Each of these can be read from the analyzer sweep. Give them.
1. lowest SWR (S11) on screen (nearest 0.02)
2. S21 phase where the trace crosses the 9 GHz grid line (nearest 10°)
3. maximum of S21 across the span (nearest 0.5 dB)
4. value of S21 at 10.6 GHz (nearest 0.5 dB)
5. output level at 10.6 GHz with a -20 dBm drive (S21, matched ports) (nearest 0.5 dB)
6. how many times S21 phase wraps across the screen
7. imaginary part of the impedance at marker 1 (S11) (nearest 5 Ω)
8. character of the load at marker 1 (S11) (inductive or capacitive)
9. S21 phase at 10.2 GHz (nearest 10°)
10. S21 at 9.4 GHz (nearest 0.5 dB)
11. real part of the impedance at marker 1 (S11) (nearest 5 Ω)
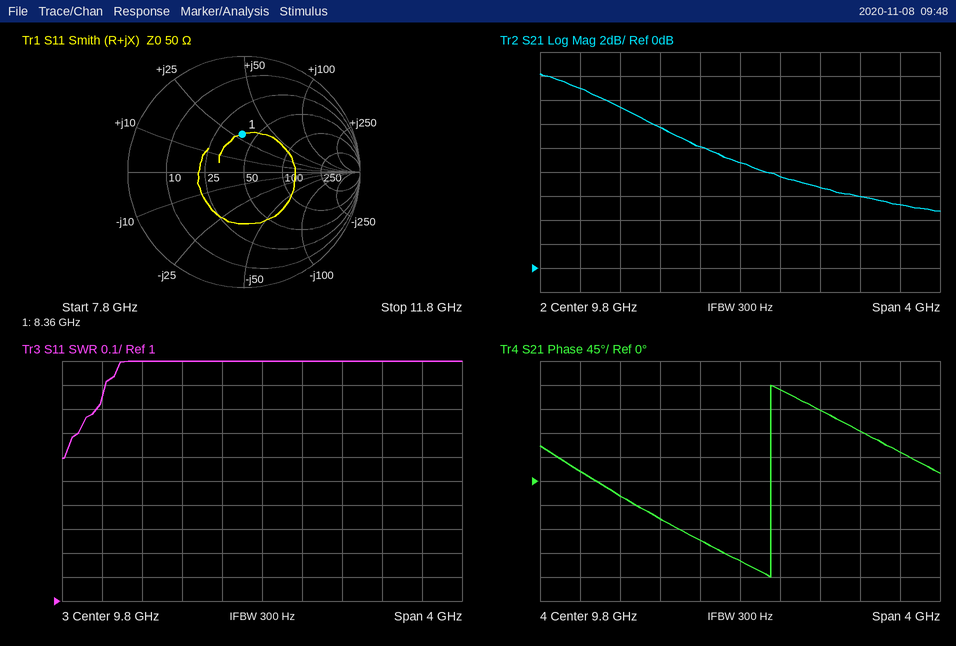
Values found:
1.60
-70°
16.0 dB
6.5 dB
-13.5 dBm
1
+30 Ω
inductive
170°
10.0 dB
40 Ω
